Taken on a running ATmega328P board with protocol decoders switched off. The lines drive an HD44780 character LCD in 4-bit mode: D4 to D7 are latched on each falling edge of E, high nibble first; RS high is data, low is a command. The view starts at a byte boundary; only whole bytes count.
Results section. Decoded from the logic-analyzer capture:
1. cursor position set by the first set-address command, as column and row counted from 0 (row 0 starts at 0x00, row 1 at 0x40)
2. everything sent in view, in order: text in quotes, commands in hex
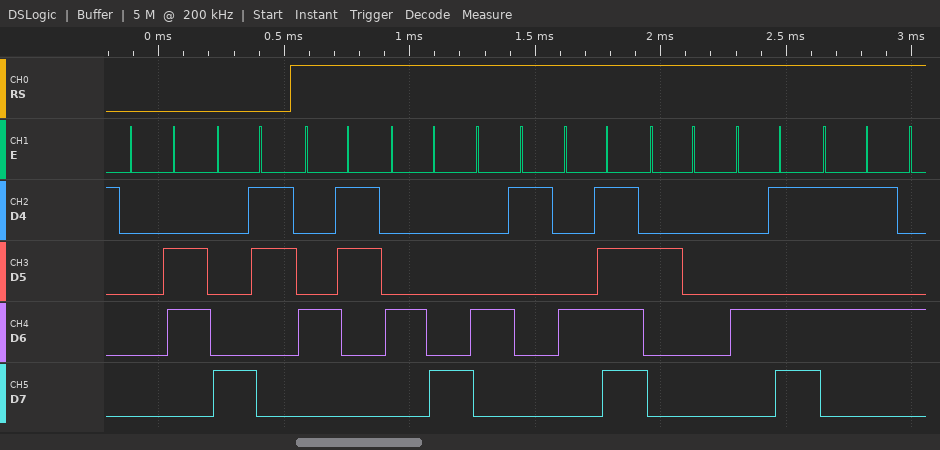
column 3, row 0
0x06 0x83 "CHAO MU"
